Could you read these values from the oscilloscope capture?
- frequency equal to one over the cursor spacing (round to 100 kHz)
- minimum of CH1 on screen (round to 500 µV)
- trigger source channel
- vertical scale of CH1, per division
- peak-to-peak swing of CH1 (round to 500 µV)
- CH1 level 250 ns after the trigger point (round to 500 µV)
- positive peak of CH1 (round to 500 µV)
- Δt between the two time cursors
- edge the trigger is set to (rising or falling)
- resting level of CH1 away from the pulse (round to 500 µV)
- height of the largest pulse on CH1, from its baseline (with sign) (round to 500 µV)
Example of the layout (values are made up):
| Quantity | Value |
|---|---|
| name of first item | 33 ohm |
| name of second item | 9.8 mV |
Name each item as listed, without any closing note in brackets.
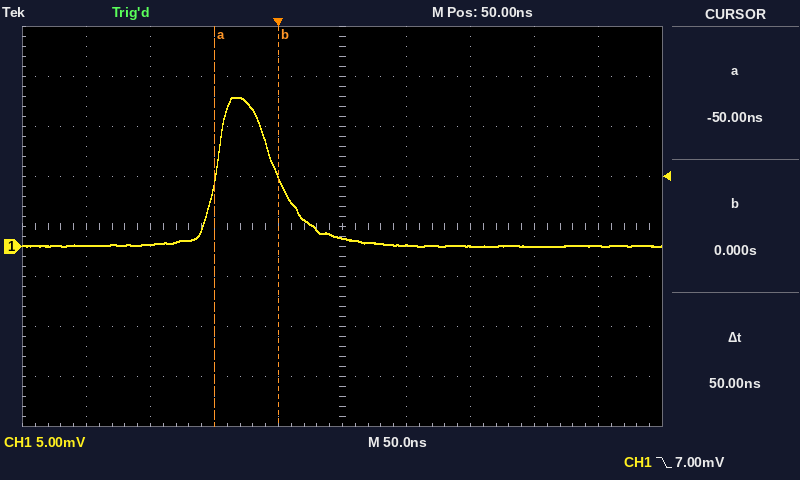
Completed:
| Quantity | Value |
|---|---|
| frequency equal to one over the cursor spacing | 20.0 MHz |
| minimum of CH1 on screen | 0.0 mV |
| trigger source channel | CH1 |
| vertical scale of CH1, per division | 5 mV |
| peak-to-peak swing of CH1 | 15.0 mV |
| CH1 level 250 ns after the trigger point | 0.0 mV |
| positive peak of CH1 | 15.0 mV |
| Δt between the two time cursors | 50 ns |
| edge the trigger is set to | falling |
| resting level of CH1 away from the pulse | 0.0 mV |
| height of the largest pulse on CH1, from its baseline (with sign) | +15.0 mV |
